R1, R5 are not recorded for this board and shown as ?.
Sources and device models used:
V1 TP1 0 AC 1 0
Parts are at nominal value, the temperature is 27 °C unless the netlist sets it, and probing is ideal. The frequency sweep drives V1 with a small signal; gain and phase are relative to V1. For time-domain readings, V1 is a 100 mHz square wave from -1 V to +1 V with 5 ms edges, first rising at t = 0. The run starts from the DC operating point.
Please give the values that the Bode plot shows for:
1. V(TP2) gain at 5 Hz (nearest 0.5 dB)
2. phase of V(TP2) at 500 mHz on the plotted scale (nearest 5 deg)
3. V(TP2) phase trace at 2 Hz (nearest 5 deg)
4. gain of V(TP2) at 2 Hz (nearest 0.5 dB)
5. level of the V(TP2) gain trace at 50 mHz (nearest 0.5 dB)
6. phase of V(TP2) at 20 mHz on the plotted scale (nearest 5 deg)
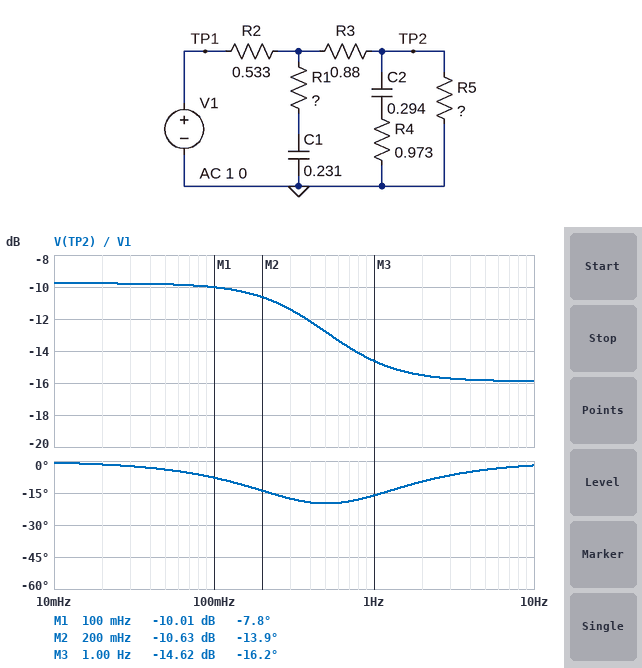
-16.0 dB
-20 deg
-10 deg
-15.5 dB
-10.0 dB
0 deg
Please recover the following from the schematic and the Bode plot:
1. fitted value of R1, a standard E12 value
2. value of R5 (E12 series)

1 Ω
0.68 Ω
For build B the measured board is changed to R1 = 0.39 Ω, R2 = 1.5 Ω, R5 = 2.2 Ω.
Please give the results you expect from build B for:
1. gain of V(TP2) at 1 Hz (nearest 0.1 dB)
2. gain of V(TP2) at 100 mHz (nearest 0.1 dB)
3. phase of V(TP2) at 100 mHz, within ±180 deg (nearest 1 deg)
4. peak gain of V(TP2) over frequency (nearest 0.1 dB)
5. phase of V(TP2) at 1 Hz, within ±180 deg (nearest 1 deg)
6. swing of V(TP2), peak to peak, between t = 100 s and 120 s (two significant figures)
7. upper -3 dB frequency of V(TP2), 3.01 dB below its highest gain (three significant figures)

-17.1 dB
-7.1 dB
-19 deg
-6.4 dB
-43 deg
960 mV
240 mHz
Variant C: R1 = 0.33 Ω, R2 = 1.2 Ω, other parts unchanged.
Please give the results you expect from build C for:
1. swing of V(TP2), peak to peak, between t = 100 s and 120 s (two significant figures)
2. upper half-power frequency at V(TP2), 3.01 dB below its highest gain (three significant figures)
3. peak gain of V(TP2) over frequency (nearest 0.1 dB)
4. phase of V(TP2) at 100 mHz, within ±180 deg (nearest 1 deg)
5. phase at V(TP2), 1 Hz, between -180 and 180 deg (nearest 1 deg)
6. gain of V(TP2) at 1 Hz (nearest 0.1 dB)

490 mV
425 mHz
-12.2 dB
-11 deg
-37 deg
-19.1 dB
